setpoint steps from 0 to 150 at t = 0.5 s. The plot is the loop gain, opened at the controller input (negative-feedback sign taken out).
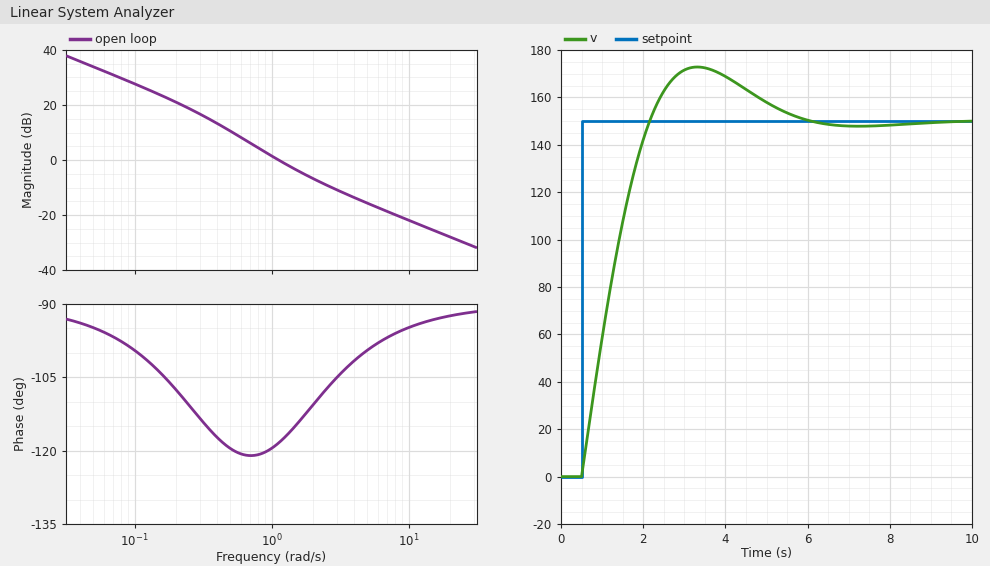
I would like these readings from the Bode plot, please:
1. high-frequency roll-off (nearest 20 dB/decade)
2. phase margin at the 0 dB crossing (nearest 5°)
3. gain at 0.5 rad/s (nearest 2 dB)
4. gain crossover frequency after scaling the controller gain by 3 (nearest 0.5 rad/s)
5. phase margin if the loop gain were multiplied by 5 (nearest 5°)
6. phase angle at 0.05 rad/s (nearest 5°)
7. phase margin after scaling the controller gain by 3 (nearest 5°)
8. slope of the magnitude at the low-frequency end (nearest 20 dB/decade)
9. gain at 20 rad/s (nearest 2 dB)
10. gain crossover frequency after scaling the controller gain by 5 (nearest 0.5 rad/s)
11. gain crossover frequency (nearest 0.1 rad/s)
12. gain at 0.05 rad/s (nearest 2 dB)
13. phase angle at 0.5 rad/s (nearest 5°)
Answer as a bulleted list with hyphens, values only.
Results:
- -20 dB/decade
- 60°
- 10 dB
- 2.5 rad/s
- 80°
- -95°
- 75°
- -20 dB/decade
- -28 dB
- 4.0 rad/s
- 1.1 rad/s
- 34 dB
- -120°
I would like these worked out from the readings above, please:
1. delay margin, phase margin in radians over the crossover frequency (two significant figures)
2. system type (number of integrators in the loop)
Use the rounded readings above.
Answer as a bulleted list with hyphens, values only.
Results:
- 0.95 s
- 1
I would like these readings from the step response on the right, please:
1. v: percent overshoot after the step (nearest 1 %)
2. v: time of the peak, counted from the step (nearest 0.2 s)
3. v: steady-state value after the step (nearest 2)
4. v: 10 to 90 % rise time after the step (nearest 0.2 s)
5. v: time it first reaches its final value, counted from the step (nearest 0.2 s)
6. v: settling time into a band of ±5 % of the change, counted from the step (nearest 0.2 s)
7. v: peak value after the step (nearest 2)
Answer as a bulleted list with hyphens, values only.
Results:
- 15 %
- 2.8 s
- 150
- 1.2 s
- 1.6 s
- 4.6 s
- 172
